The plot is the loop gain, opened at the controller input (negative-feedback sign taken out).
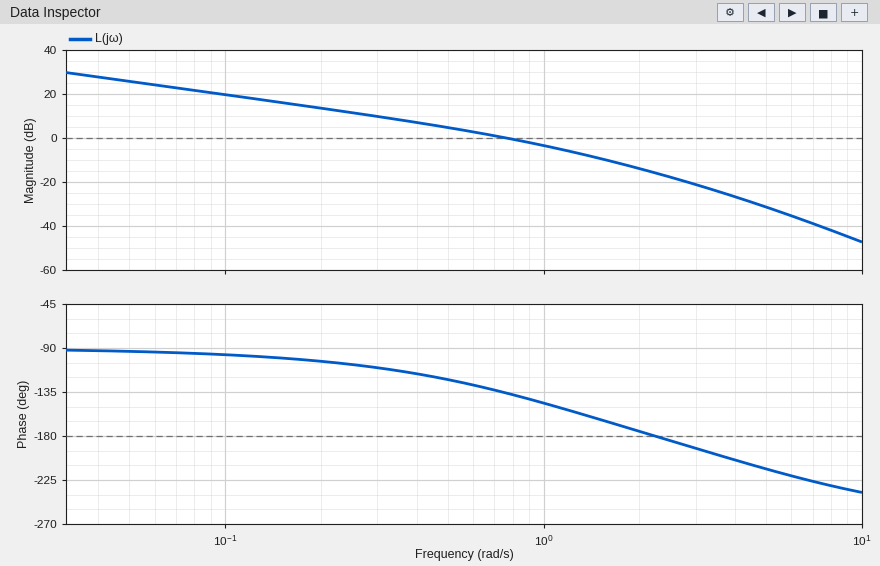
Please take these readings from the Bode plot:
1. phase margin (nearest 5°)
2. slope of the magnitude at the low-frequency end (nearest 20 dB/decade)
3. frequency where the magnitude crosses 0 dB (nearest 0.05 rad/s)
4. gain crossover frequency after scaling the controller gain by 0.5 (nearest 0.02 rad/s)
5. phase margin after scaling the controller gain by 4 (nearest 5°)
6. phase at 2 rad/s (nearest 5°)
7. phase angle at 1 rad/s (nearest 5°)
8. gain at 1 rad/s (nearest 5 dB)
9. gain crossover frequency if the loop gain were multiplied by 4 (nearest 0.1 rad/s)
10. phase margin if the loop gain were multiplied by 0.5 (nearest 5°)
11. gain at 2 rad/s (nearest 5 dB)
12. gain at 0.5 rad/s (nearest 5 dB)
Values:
45°
-20 dB/decade
0.75 rad/s
0.44 rad/s
10°
-175°
-145°
-5 dB
1.8 rad/s
60°
-15 dB
5 dB
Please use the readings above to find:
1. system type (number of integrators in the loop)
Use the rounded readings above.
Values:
1
